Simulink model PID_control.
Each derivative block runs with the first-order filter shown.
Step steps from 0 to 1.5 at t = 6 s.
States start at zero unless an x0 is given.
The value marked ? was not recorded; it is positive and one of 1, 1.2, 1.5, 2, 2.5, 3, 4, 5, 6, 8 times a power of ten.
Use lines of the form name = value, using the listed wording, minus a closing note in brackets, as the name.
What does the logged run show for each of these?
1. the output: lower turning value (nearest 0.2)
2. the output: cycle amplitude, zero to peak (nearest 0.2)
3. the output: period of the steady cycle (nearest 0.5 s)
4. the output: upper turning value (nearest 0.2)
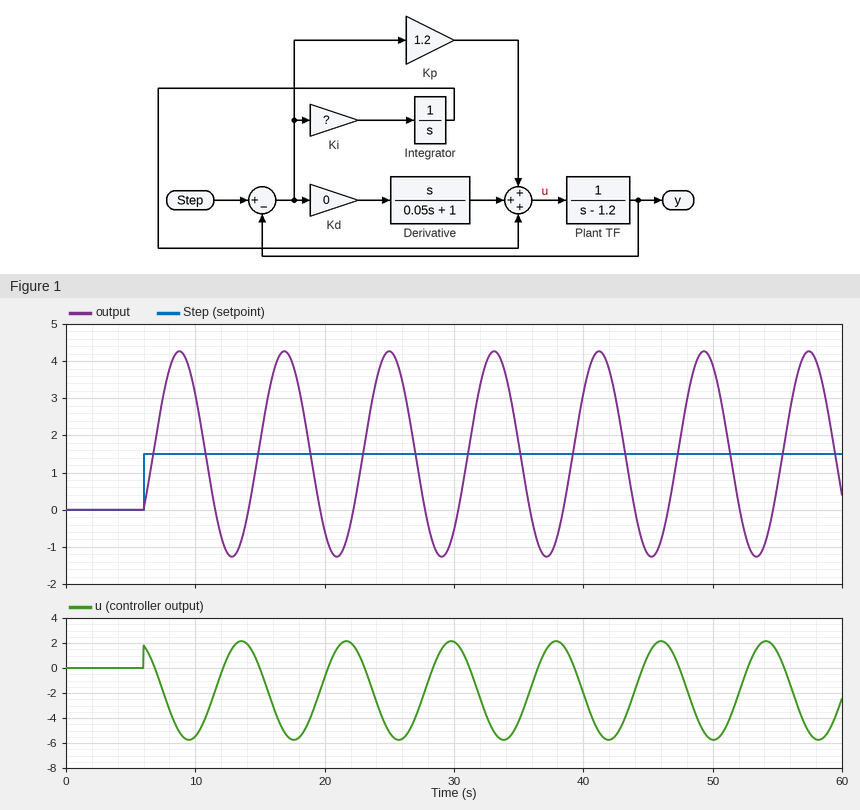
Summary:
the output: lower turning value = -1.2
the output: cycle amplitude, zero to peak = 2.8
the output: period of the steady cycle = 8.0 s
the output: upper turning value = 4.2
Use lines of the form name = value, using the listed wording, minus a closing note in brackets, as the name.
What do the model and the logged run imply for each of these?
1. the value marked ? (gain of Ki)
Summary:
the value marked ? = 0.6
